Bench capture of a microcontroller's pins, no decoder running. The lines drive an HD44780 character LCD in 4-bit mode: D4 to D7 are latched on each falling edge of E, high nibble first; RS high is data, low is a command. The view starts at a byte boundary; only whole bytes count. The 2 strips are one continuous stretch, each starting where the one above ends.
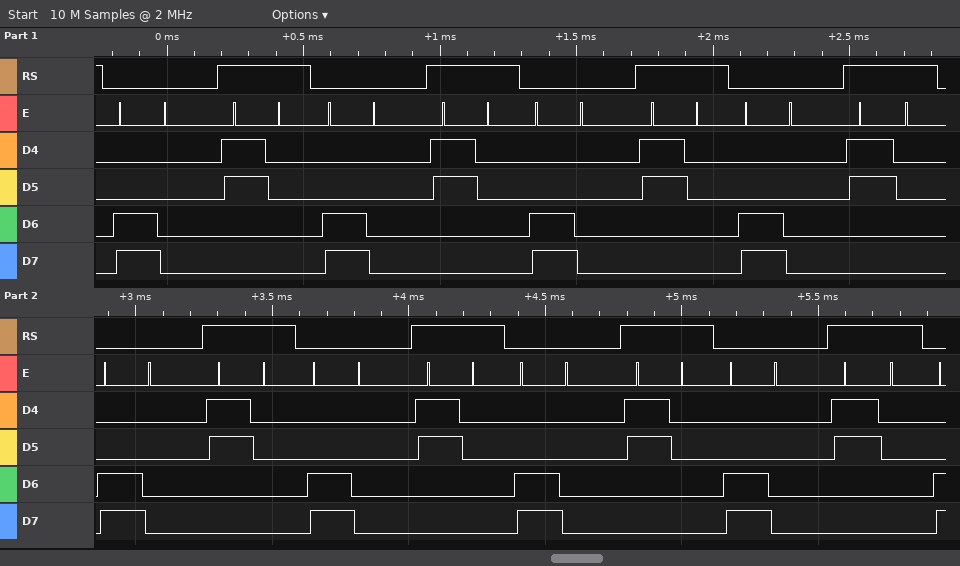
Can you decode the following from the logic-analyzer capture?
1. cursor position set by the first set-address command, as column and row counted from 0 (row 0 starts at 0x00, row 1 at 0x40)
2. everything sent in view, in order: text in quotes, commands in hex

column 0, row 1
0xC0 "0" 0xC0 "0" 0xC0 "0" 0xC0 "0" 0xC0 "0" 0xC0 "0" 0xC0 "0" 0xC0 "0"
